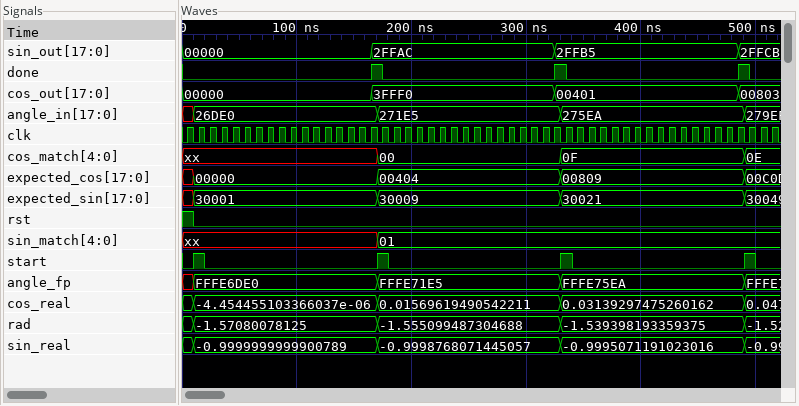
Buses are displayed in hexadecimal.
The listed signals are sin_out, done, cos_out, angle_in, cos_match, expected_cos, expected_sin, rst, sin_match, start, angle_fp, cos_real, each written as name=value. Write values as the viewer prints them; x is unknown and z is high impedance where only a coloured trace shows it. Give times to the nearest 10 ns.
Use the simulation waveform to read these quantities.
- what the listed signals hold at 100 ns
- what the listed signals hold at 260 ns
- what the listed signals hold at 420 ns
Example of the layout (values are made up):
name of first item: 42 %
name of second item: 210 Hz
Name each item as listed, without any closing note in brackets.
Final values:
what the listed signals hold at 100 ns: sin_out=00000, done=0, cos_out=00000, angle_in=26DE0, cos_match=xx, expected_cos=00000, expected_sin=30001, rst=0, sin_match=xx, start=0, angle_fp=FFFE6DE0, cos_real=-4.454455103366037e-06
what the listed signals hold at 260 ns: sin_out=2FFAC, done=0, cos_out=3FFF0, angle_in=271E5, cos_match=00, expected_cos=00404, expected_sin=30009, rst=0, sin_match=01, start=0, angle_fp=FFFE71E5, cos_real=0.01569619490542211
what the listed signals hold at 420 ns: sin_out=2FFB5, done=0, cos_out=00401, angle_in=275EA, cos_match=0F, expected_cos=00809, expected_sin=30021, rst=0, sin_match=01, start=0, angle_fp=FFFE75EA, cos_real=0.03139297475260162
